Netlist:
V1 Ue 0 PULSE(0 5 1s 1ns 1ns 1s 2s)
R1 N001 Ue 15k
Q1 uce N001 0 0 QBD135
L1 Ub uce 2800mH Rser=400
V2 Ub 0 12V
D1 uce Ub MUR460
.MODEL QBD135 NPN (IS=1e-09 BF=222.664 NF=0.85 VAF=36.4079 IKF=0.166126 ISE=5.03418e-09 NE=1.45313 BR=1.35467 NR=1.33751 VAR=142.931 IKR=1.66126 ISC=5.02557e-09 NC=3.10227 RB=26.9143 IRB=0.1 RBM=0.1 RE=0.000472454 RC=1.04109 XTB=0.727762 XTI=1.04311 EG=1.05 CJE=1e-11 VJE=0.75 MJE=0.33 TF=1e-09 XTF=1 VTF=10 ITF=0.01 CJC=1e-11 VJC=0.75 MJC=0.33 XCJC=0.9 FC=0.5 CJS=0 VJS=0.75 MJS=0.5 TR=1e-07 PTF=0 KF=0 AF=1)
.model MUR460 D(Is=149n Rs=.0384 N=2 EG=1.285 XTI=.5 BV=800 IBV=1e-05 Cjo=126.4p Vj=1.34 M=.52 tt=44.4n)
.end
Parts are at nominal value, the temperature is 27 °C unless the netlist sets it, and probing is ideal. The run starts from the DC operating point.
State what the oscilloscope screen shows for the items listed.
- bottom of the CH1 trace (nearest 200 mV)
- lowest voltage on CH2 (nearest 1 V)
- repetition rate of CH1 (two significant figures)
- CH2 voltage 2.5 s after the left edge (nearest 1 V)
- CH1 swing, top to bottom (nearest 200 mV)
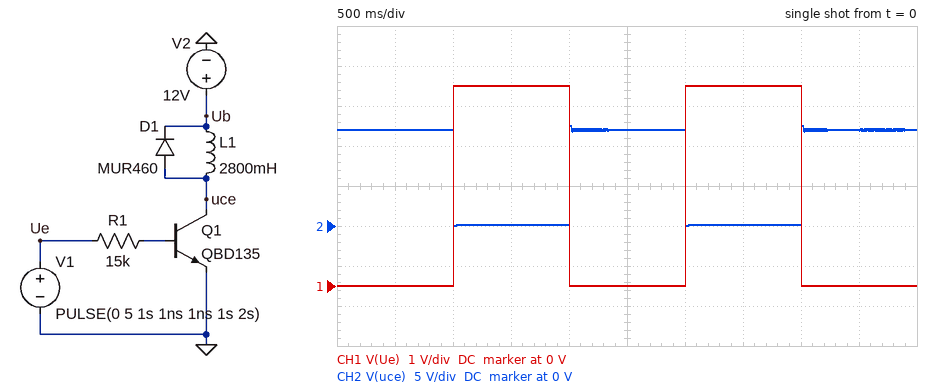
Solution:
0 V
0 V
500 mHz
12 V
5.0 V
